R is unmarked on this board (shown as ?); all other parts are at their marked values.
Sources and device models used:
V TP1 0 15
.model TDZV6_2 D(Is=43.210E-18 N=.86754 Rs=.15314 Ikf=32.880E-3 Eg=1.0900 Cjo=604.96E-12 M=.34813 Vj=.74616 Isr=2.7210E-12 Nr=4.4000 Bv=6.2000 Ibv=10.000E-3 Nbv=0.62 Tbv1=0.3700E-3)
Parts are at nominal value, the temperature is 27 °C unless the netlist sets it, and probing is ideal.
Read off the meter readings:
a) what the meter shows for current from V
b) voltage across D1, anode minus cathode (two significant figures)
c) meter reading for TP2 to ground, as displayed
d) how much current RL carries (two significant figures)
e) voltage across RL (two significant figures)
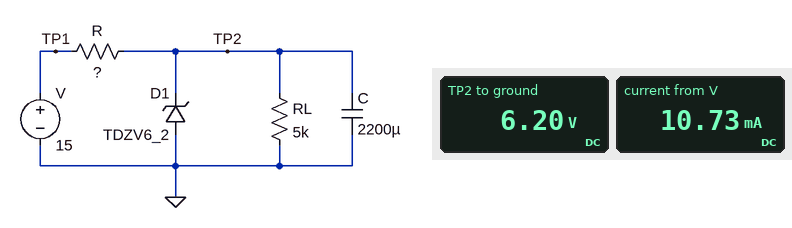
10.73 mA
-6.2 V
6.20 V
1.2 mA
6.2 V
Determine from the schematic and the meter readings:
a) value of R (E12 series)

820 Ω
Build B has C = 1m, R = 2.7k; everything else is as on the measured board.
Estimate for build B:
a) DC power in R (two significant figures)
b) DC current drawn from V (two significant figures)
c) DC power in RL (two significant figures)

29 mW
3.3 mA
7.6 mW
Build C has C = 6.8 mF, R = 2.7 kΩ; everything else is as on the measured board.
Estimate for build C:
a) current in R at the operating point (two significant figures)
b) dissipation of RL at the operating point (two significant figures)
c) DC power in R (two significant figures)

3.3 mA
7.6 mW
29 mW
